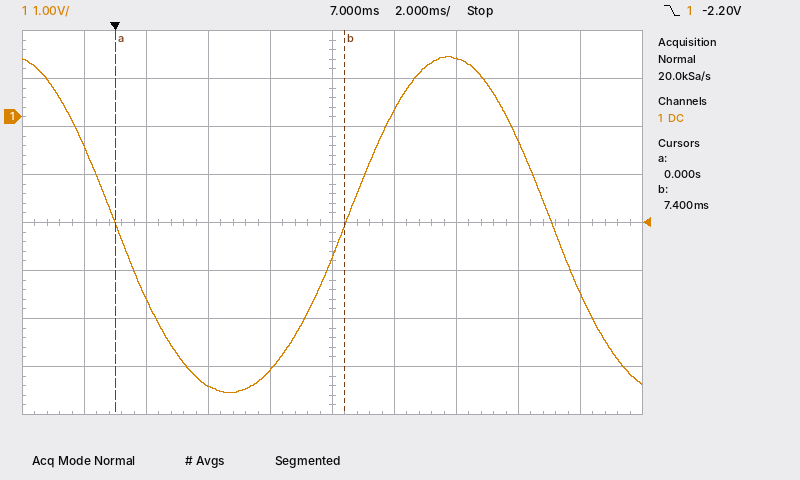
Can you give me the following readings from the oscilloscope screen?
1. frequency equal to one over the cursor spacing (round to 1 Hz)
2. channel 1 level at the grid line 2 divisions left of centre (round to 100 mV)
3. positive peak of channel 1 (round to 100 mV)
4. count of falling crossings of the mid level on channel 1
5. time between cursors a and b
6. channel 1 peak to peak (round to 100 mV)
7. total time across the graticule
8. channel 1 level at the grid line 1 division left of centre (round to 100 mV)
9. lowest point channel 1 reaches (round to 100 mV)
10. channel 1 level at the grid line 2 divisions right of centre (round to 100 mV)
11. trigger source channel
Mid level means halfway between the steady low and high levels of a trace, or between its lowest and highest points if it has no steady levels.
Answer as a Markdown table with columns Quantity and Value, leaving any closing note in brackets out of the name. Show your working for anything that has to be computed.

| Quantity | Value |
|---|---|
| frequency equal to one over the cursor spacing | 1 / 7.4 ms ≈ 135 Hz |
| channel 1 level at the grid line 2 divisions left of centre | -5.6 V |
| positive peak of channel 1 | 1.3 V |
| count of falling crossings of the mid level on channel 1 | 2 |
| time between cursors a and b | 7.4 ms − (0 s) = 7.4 ms |
| channel 1 peak to peak | 1.3 V − (-5.7 V) = 7.0 V |
| total time across the graticule | 20 ms |
| channel 1 level at the grid line 1 division left of centre | -5.3 V |
| lowest point channel 1 reaches | -5.7 V |
| channel 1 level at the grid line 2 divisions right of centre | 1.2 V |
| trigger source channel | channel 1 |
